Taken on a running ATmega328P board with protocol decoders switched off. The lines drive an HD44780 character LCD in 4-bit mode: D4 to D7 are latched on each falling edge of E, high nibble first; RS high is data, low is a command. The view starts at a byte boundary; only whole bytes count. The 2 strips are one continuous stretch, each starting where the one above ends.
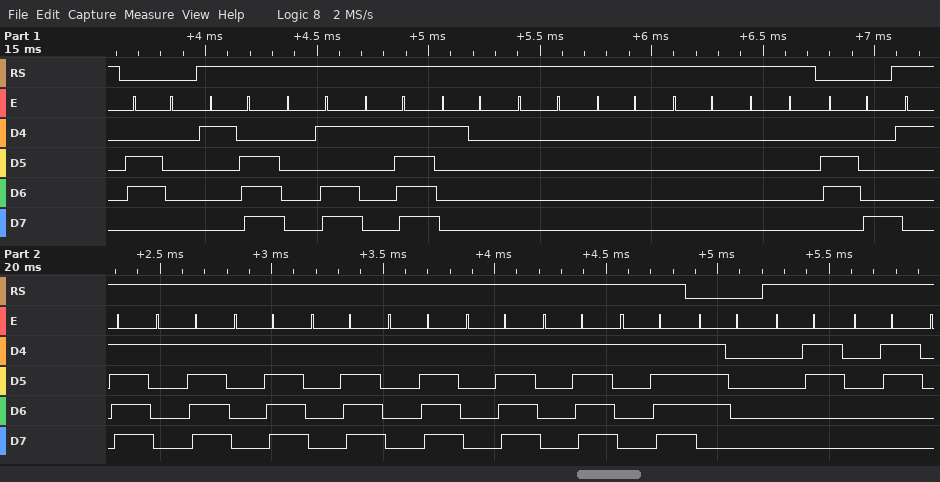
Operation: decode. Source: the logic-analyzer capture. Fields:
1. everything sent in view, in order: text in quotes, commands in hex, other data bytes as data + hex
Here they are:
0x60 data 1E 0D 1F 10 00 00 00 00 0x68 data 1F 1F 1F 1F 1F 1F 1F 1F 0x70 data 03 03
